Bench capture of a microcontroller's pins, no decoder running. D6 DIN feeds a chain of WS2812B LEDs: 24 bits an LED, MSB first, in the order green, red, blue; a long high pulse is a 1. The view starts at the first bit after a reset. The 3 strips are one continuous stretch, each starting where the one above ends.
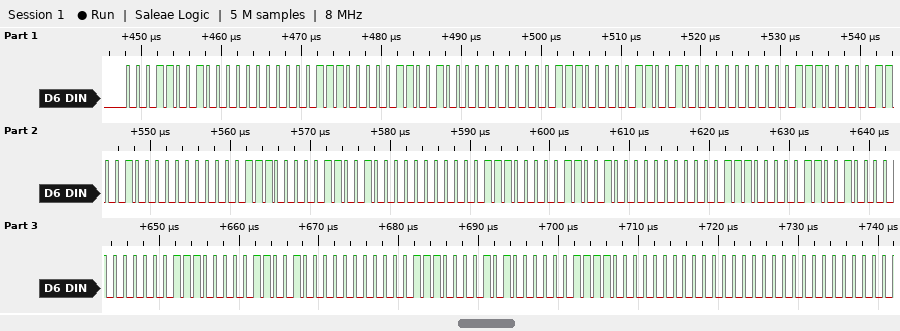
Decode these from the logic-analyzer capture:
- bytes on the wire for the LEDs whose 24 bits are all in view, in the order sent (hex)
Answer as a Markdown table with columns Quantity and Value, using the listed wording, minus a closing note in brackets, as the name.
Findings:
| Quantity | Value |
|---|---|
| bytes on the wire for the LEDs whose 24 bits are all in view, in the order sent | 19 00 1C 19 00 1C 19 00 1C 19 00 1C 19 00 1C 19 00 1C 19 00 1C 19 00 1C 28 1E 00 |
